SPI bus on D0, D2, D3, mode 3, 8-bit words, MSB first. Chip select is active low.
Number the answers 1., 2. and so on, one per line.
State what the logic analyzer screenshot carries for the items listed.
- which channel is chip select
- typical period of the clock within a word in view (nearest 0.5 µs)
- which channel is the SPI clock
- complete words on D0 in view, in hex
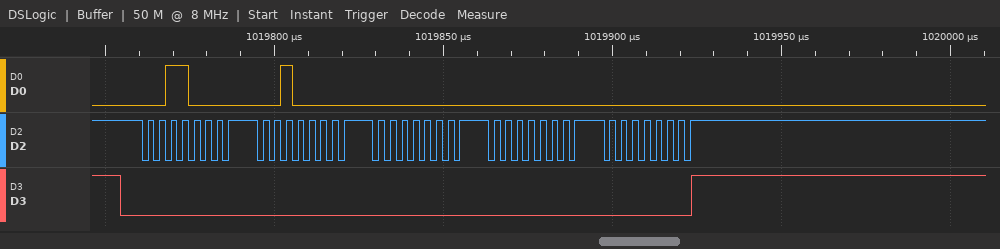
1. D3
2. 3.5 µs
3. D2
4. 30, 20, 00, 00, 00
